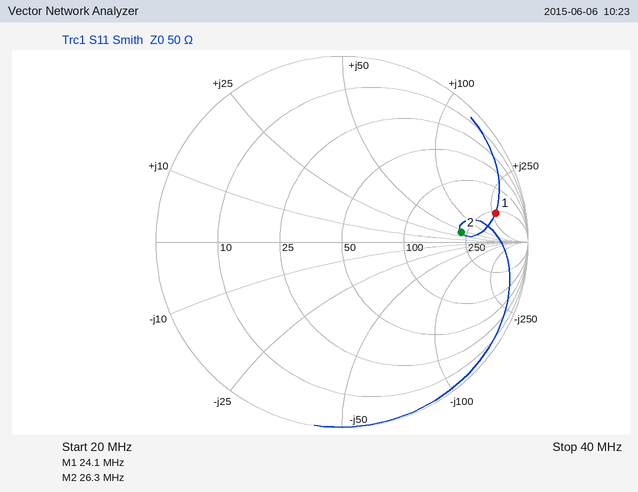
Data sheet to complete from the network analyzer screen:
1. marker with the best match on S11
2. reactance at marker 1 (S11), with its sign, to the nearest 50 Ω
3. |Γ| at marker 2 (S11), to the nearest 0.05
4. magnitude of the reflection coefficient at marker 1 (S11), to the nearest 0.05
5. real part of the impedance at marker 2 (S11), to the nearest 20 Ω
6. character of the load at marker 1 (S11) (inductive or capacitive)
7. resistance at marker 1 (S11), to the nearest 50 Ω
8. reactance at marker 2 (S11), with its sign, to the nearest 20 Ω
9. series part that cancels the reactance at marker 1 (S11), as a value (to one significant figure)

marker 2
+300 Ω
0.65
0.85
220 Ω
inductive
250 Ω
+40 Ω
20 pF
